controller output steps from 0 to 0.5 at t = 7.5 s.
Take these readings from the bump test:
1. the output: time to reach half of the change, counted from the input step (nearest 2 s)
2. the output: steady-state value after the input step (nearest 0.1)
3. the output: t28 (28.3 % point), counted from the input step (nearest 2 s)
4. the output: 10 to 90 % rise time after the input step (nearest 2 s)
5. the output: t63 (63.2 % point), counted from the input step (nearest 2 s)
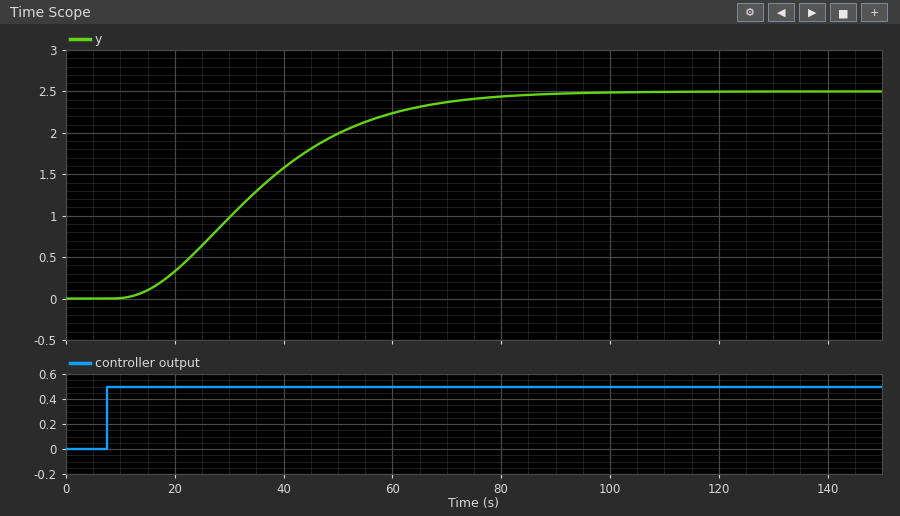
26 s
2.5
18 s
42 s
32 s
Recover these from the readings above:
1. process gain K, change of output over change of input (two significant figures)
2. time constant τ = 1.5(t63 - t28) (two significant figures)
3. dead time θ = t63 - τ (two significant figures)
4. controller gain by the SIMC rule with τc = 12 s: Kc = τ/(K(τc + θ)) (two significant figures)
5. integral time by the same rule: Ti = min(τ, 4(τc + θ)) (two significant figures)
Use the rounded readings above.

5.0
21 s
11 s
0.18
21 s
